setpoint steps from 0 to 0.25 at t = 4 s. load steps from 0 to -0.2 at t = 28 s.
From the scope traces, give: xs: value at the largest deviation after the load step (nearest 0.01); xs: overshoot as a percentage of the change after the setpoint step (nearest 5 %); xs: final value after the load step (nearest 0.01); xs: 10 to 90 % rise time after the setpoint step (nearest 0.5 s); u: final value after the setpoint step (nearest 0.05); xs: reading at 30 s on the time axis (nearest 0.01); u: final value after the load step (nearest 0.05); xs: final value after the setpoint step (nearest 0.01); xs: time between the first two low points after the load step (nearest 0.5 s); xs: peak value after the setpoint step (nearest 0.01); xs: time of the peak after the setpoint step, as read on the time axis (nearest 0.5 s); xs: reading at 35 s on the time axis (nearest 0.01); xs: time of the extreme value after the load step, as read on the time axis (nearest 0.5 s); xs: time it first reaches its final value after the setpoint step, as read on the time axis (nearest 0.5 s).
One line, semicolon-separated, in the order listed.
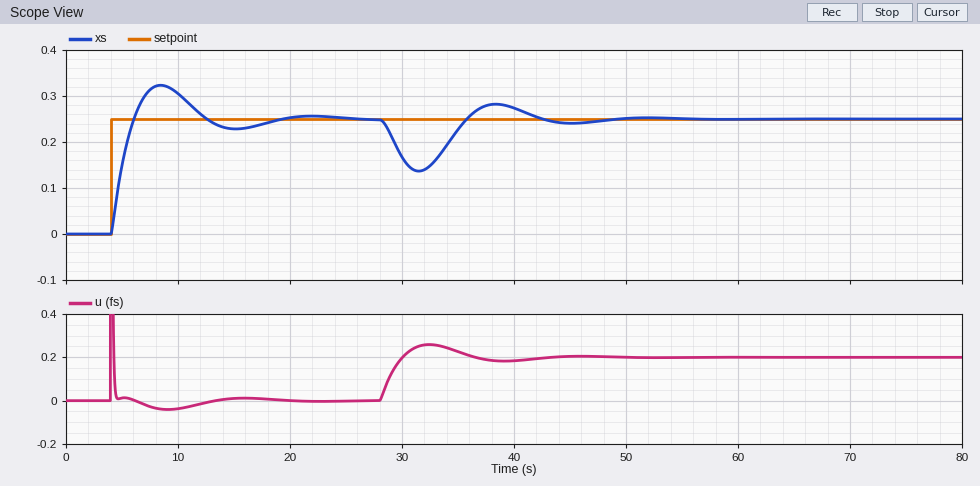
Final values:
0.14; 30 %; 0.25; 1.5 s; 0.00; 0.17; 0.20; 0.25; 13.5 s; 0.32; 8.5 s; 0.23; 31.5 s; 6.0 s
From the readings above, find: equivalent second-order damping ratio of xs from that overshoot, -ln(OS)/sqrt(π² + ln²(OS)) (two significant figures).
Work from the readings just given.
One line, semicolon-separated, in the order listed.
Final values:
0.36
